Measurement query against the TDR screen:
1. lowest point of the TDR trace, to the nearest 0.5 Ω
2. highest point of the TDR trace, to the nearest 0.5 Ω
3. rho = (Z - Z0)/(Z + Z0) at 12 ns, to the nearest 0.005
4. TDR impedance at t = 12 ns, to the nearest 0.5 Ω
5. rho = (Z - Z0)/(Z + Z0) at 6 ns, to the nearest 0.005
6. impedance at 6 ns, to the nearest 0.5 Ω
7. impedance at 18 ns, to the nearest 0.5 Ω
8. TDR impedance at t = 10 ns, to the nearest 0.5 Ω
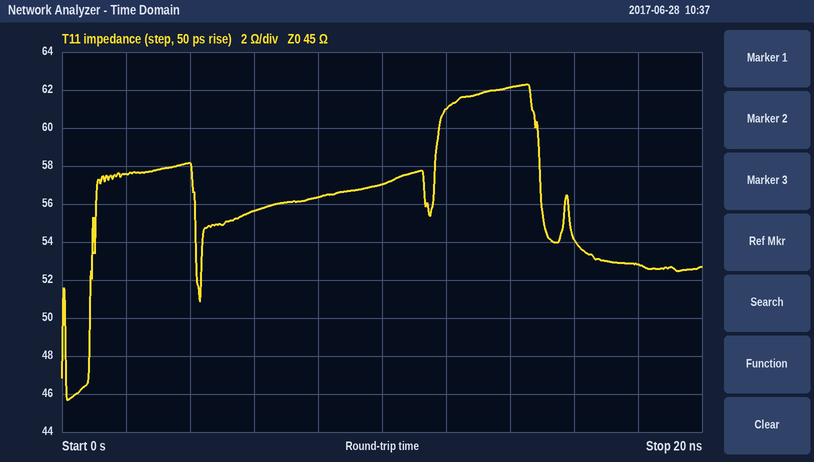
45.5 Ω
62.5 Ω
+0.150
61.0 Ω
+0.105
55.5 Ω
53.0 Ω
57.0 Ω
